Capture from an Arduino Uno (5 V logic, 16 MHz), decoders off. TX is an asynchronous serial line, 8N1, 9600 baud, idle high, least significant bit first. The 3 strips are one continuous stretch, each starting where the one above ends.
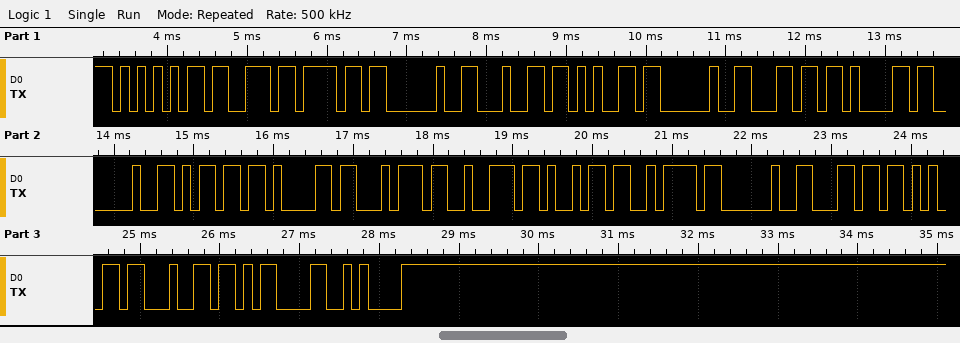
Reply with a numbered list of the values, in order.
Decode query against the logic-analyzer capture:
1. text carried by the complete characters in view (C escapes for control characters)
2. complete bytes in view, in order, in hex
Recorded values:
1. "Uso de la matriz led\r\n"
2. 55 73 6F 20 64 65 20 6C 61 20 6D 61 74 72 69 7A 20 6C 65 64 0D 0A
